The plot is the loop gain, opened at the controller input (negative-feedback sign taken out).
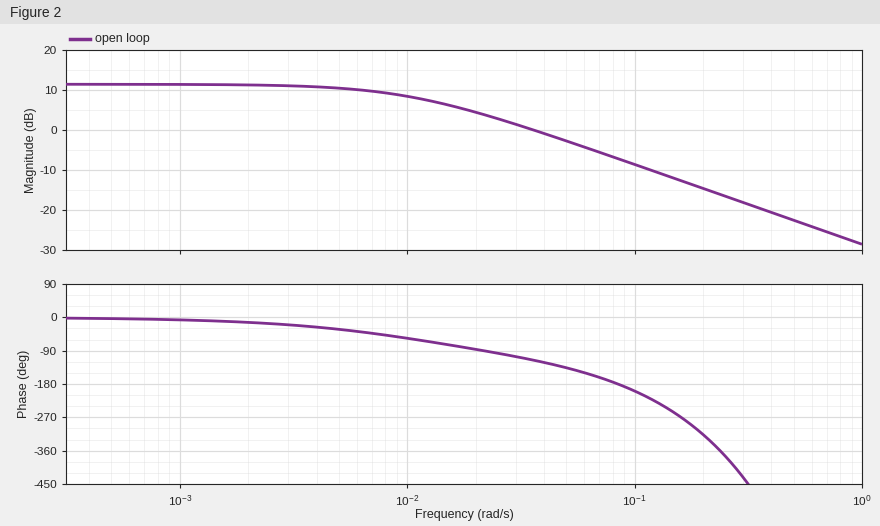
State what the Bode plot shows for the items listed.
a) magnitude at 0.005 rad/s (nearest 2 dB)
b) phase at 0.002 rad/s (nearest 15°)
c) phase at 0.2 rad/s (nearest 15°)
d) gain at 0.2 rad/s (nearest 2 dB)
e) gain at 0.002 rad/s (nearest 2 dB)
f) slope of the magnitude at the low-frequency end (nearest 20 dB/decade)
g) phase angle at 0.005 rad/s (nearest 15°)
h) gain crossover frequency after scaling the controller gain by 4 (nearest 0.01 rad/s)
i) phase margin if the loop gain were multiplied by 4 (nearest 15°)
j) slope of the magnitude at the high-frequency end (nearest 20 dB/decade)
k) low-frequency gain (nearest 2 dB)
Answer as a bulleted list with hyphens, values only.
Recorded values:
- 10 dB
- -15°
- -315°
- -14 dB
- 12 dB
- 0 dB/decade
- -30°
- 0.15 rad/s
- -75°
- -20 dB/decade
- 12 dB
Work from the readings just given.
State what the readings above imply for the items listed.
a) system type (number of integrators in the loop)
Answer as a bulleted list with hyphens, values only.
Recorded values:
- 0
